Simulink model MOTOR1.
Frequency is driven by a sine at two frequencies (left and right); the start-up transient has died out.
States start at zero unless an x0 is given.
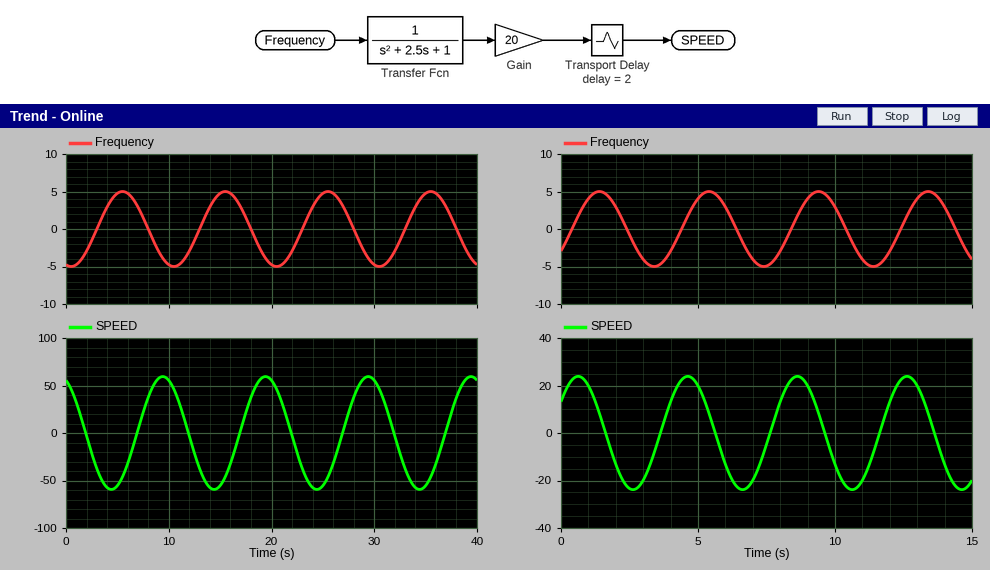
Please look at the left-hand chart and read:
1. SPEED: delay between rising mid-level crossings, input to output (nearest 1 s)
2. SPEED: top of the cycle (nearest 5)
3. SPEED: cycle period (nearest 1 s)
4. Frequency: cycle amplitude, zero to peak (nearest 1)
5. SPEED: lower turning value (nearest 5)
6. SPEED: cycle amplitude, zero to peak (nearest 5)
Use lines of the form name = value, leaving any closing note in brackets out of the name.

SPEED: delay between rising mid-level crossings, input to output = 4 s
SPEED: top of the cycle = 60
SPEED: cycle period = 10 s
Frequency: cycle amplitude, zero to peak = 5
SPEED: lower turning value = -60
SPEED: cycle amplitude, zero to peak = 60
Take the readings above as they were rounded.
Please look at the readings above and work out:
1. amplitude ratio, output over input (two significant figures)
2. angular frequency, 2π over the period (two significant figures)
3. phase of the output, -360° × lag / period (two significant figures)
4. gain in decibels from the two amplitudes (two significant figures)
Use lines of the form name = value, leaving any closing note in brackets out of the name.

amplitude ratio, output over input = 12
angular frequency, 2π over the period = 0.63 rad/s
phase of the output, -360° × lag / period = -140°
gain in decibels from the two amplitudes = 22 dB
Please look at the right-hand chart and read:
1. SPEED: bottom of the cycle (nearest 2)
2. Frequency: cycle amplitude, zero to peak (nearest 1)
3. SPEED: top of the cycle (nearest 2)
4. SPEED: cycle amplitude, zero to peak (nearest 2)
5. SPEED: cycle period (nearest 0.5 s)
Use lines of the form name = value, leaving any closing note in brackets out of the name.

SPEED: bottom of the cycle = -24
Frequency: cycle amplitude, zero to peak = 5
SPEED: top of the cycle = 24
SPEED: cycle amplitude, zero to peak = 24
SPEED: cycle period = 4.0 s
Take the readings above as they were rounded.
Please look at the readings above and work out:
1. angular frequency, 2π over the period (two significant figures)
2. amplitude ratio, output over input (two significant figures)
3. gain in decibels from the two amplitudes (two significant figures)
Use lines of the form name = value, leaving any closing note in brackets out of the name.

angular frequency, 2π over the period = 1.6 rad/s
amplitude ratio, output over input = 4.8
gain in decibels from the two amplitudes = 14 dB
